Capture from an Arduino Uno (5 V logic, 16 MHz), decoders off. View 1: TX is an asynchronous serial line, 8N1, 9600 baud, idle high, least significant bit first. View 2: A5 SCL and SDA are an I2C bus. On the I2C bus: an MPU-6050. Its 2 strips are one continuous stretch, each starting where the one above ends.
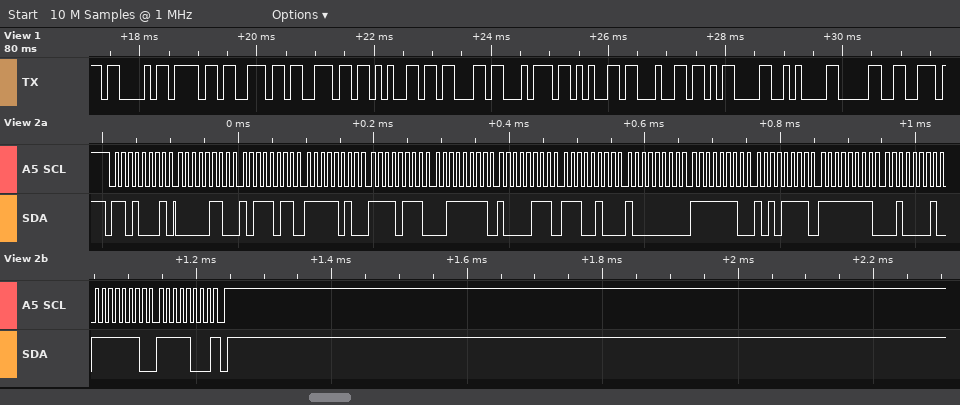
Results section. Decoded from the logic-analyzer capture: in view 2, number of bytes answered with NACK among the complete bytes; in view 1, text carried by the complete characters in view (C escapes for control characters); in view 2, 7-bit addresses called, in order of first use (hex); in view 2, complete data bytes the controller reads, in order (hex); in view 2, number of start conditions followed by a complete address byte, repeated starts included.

1
"Connected\r\n0"
0x68
06 BB FA F7 3F 87 E4 80 FE AF FF 21 FE F8
1
